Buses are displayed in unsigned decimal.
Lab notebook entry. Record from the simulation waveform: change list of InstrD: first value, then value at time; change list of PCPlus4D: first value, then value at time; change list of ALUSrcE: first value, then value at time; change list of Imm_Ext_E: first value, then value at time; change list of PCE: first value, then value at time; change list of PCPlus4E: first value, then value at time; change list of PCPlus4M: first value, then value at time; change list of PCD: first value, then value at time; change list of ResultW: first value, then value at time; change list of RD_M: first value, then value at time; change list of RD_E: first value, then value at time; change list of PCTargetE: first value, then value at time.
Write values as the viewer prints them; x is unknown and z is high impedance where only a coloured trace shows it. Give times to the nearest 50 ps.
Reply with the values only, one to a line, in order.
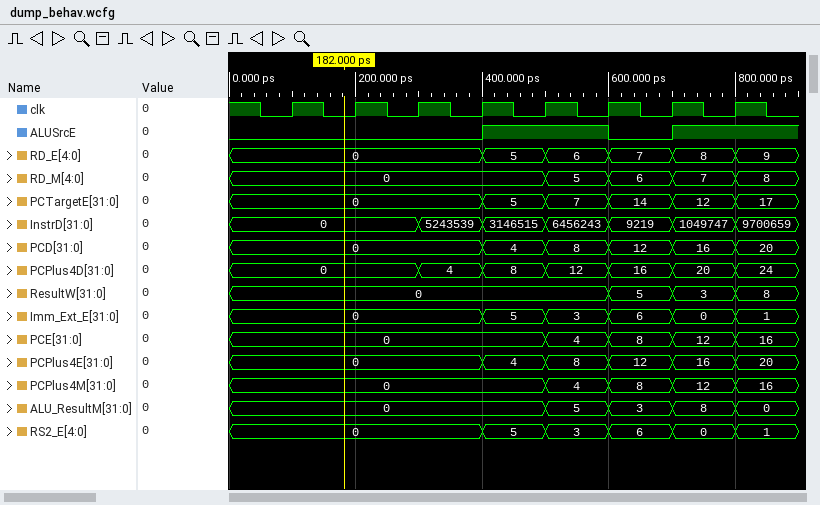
0, 5243539 at 300 ps, 3146515 at 400 ps, 6456243 at 500 ps, 9219 at 600 ps, 1049747 at 700 ps, 9700659 at 800 ps
0, 4 at 300 ps, 8 at 400 ps, 12 at 500 ps, 16 at 600 ps, 20 at 700 ps, 24 at 800 ps
0, 1 at 400 ps, 0 at 600 ps, 1 at 700 ps
0, 5 at 400 ps, 3 at 500 ps, 6 at 600 ps, 0 at 700 ps, 1 at 800 ps
0, 4 at 500 ps, 8 at 600 ps, 12 at 700 ps, 16 at 800 ps
0, 4 at 400 ps, 8 at 500 ps, 12 at 600 ps, 16 at 700 ps, 20 at 800 ps
0, 4 at 500 ps, 8 at 600 ps, 12 at 700 ps, 16 at 800 ps
0, 4 at 400 ps, 8 at 500 ps, 12 at 600 ps, 16 at 700 ps, 20 at 800 ps
0, 5 at 600 ps, 3 at 700 ps, 8 at 800 ps
0, 5 at 500 ps, 6 at 600 ps, 7 at 700 ps, 8 at 800 ps
0, 5 at 400 ps, 6 at 500 ps, 7 at 600 ps, 8 at 700 ps, 9 at 800 ps
0, 5 at 400 ps, 7 at 500 ps, 14 at 600 ps, 12 at 700 ps, 17 at 800 ps
